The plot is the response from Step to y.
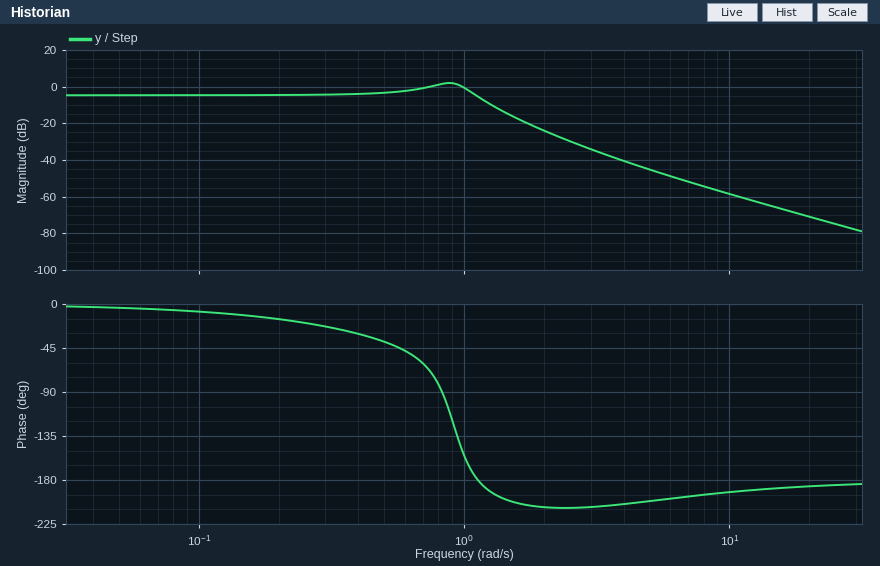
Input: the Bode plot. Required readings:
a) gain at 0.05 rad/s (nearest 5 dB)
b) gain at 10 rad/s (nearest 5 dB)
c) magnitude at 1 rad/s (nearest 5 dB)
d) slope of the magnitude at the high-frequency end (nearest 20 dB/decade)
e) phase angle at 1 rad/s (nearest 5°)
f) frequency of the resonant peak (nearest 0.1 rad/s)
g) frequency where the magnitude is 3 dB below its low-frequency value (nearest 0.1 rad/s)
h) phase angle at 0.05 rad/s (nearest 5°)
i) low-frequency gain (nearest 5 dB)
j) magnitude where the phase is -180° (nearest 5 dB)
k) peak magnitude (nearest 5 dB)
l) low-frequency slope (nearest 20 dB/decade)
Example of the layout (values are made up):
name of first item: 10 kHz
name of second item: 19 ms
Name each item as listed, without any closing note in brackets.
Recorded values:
gain at 0.05 rad/s: -5 dB
gain at 10 rad/s: -60 dB
magnitude at 1 rad/s: 0 dB
slope of the magnitude at the high-frequency end: -40 dB/decade
phase angle at 1 rad/s: -155°
frequency of the resonant peak: 0.9 rad/s
frequency where the magnitude is 3 dB below its low-frequency value: 1.2 rad/s
phase angle at 0.05 rad/s: -5°
low-frequency gain: -5 dB
magnitude where the phase is -180°: -5 dB
peak magnitude: 0 dB
low-frequency slope: 0 dB/decade
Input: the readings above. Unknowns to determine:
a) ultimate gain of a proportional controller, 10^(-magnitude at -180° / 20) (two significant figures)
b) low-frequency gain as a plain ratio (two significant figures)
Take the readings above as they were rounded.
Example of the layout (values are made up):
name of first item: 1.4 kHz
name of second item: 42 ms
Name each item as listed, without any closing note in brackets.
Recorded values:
ultimate gain of a proportional controller, 10^(-magnitude at -180° / 20): 1.8
low-frequency gain as a plain ratio: 0.56
